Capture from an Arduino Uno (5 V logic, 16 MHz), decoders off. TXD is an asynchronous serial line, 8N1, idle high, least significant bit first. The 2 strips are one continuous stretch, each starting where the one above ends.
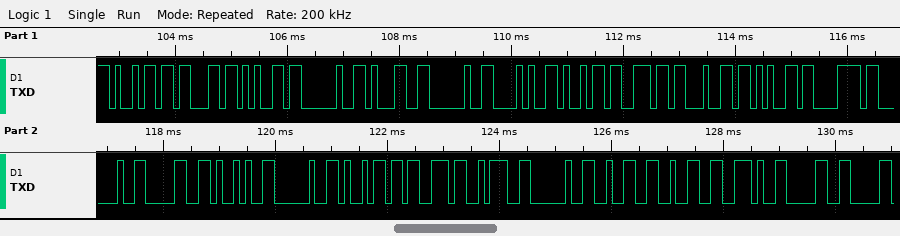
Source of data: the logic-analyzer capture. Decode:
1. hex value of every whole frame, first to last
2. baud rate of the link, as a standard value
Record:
69 63 65 20 31 20 28 69 6E 64 65 78 20 30 29 20 69 73 3A 20 32 32 2E 30
9600 baud
